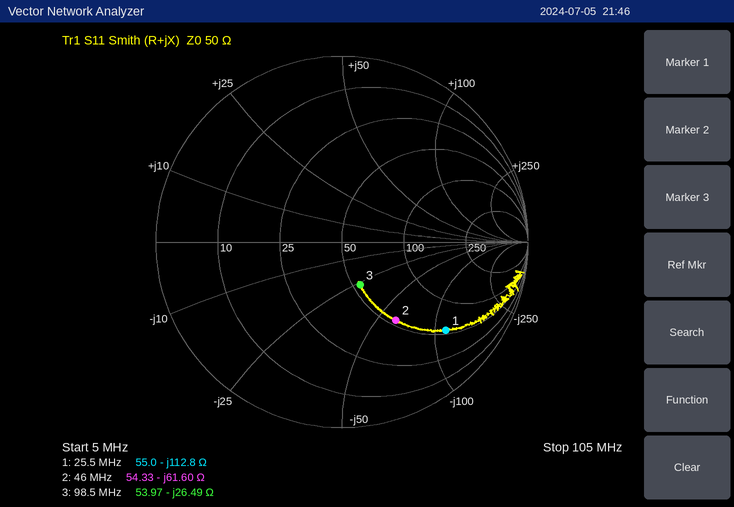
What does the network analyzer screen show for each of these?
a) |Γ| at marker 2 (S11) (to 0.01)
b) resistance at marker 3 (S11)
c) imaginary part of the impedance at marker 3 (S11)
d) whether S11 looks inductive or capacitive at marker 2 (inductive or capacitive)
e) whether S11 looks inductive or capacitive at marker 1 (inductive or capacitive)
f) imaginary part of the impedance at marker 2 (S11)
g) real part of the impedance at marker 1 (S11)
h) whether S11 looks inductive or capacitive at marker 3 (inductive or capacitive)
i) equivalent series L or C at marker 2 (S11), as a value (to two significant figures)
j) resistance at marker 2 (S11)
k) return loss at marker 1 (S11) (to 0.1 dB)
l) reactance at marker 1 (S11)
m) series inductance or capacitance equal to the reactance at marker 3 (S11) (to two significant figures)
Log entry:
0.51
53.97 Ω
-26.49 Ω
capacitive
capacitive
-61.60 Ω
55.0 Ω
capacitive
56 pF
54.33 Ω
2.7 dB
-112.8 Ω
61 pF
